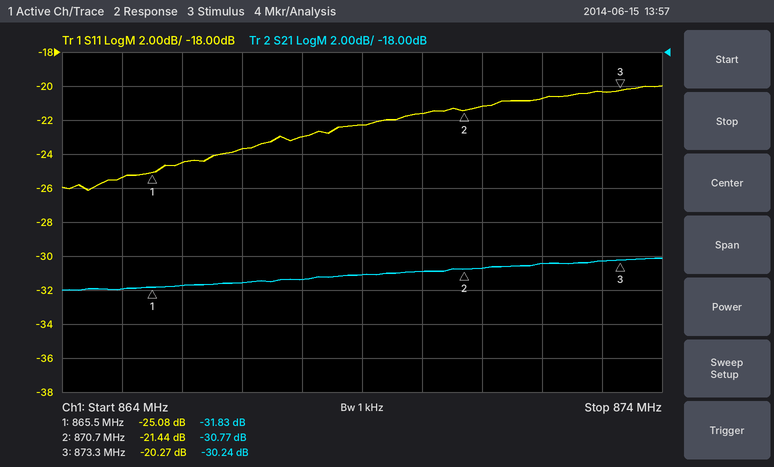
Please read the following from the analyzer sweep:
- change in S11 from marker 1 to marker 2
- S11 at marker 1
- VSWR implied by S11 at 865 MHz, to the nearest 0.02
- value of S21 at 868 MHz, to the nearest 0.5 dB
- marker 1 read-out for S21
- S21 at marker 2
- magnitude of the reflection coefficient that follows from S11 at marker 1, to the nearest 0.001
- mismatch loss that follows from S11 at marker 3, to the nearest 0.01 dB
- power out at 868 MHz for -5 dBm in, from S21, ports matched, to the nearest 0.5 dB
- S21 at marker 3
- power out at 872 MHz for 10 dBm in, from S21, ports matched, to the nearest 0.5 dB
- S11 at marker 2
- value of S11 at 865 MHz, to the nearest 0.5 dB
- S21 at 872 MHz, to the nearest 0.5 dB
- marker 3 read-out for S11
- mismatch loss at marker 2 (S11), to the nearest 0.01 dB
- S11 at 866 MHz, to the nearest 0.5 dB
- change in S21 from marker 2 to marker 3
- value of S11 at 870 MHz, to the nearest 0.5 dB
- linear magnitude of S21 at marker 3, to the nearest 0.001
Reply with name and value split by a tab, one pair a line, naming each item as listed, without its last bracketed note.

change in S11 from marker 1 to marker 2	3.64 dB
S11 at marker 1	-25.08 dB
VSWR implied by S11 at 865 MHz, to the nearest 0.02	1.12
value of S21 at 868 MHz, to the nearest 0.5 dB	-31.5 dB
marker 1 read-out for S21	-31.83 dB
S21 at marker 2	-30.77 dB
magnitude of the reflection coefficient that follows from S11 at marker 1, to the nearest 0.001	0.056
mismatch loss that follows from S11 at marker 3, to the nearest 0.01 dB	0.04 dB
power out at 868 MHz for -5 dBm in, from S21, ports matched, to the nearest 0.5 dB	-36.5 dBm
S21 at marker 3	-30.24 dB
power out at 872 MHz for 10 dBm in, from S21, ports matched, to the nearest 0.5 dB	-20.5 dBm
S11 at marker 2	-21.44 dB
value of S11 at 865 MHz, to the nearest 0.5 dB	-25.5 dB
S21 at 872 MHz, to the nearest 0.5 dB	-30.5 dB
marker 3 read-out for S11	-20.27 dB
mismatch loss at marker 2 (S11), to the nearest 0.01 dB	0.03 dB
S11 at 866 MHz, to the nearest 0.5 dB	-24.5 dB
change in S21 from marker 2 to marker 3	0.53 dB
value of S11 at 870 MHz, to the nearest 0.5 dB	-21.5 dB
linear magnitude of S21 at marker 3, to the nearest 0.001	0.031
